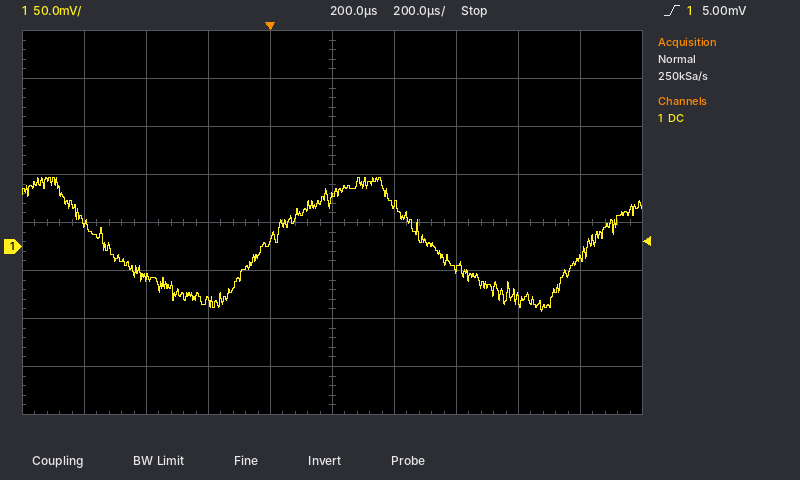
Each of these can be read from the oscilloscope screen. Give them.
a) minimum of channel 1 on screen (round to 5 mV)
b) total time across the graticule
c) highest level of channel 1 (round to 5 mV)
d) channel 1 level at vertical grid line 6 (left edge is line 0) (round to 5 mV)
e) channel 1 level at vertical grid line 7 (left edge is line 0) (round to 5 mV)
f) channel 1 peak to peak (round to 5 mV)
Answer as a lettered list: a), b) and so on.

a) -70 mV
b) 2 ms
c) 70 mV
d) 45 mV
e) -25 mV
f) 140 mV
